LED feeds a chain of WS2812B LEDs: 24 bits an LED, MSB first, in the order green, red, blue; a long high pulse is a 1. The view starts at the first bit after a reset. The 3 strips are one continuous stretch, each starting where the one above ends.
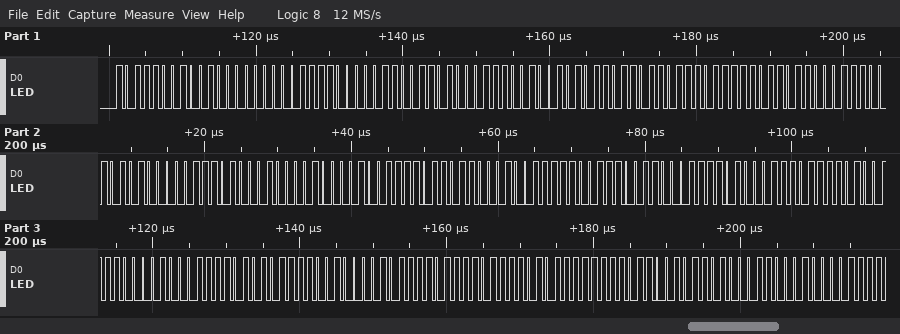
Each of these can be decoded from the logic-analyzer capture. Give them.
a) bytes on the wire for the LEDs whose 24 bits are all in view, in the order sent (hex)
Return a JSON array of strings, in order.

["B9 20 0F 06 68 E4 AD B7 7D B1 CA 83 A2 10 9E D8 9F 39 8F 47 7A 70 8F 57 90 BD EF 5F EC B4"]
